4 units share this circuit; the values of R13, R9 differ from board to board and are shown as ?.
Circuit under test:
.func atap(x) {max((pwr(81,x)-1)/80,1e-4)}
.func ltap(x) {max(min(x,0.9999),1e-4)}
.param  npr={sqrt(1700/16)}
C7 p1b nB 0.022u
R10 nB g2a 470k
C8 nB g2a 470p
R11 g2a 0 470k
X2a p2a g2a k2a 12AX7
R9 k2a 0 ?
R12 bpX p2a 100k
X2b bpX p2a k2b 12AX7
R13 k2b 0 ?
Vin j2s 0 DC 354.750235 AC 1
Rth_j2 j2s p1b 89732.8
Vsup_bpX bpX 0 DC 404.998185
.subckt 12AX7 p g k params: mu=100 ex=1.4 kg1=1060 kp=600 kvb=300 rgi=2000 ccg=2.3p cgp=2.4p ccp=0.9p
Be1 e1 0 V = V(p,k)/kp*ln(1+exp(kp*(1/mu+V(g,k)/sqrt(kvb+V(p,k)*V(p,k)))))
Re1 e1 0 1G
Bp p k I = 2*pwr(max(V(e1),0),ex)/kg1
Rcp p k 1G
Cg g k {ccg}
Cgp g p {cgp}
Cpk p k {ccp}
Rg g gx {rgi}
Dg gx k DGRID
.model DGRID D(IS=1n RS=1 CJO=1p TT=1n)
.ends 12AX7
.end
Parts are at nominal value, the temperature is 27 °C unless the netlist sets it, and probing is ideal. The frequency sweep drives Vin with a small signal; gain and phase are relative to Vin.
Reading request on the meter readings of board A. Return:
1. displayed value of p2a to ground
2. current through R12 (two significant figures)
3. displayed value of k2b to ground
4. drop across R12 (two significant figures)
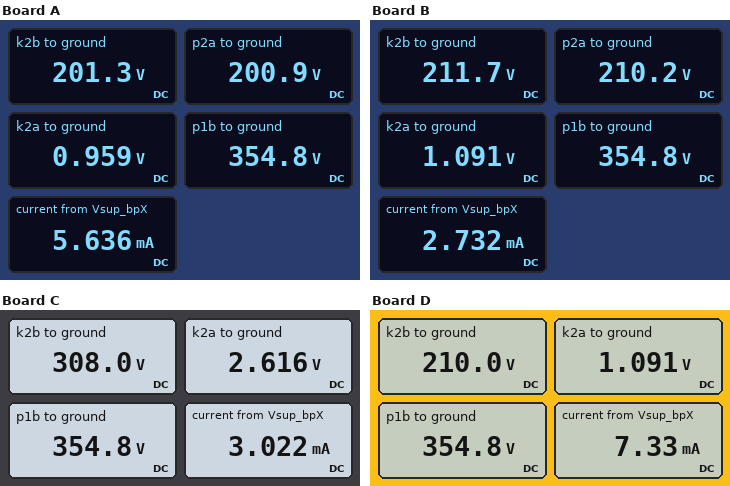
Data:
200.9 V
2.0 mA
201.3 V
200 V
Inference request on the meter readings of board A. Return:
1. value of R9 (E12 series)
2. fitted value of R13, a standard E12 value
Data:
470 Ω
56 kΩ
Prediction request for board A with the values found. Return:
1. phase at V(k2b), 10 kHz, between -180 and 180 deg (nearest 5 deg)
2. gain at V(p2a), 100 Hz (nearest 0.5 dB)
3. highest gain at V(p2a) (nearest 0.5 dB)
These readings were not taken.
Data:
155 deg
27.5 dB
31.0 dB
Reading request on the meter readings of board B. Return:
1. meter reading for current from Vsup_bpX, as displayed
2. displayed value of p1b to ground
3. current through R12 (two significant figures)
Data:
2.732 mA
354.8 V
1.9 mA
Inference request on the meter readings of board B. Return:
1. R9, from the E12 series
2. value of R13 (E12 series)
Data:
560 Ω
270 kΩ
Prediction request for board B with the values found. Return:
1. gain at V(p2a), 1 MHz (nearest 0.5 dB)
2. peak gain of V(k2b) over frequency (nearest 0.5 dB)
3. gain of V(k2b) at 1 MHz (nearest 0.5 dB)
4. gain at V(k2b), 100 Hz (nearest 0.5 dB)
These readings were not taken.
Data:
-3.0 dB
30.5 dB
-3.5 dB
27.0 dB
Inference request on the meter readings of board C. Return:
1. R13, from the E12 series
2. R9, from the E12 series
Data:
150 kΩ
2.7 kΩ
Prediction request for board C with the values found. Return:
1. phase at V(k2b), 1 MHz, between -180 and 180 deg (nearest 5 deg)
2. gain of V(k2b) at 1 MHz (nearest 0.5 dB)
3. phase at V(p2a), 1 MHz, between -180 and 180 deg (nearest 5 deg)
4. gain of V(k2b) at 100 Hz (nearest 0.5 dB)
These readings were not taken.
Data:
85 deg
-4.0 dB
85 deg
20.0 dB
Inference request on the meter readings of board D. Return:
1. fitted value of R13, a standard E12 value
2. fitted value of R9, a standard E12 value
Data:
39 kΩ
560 Ω
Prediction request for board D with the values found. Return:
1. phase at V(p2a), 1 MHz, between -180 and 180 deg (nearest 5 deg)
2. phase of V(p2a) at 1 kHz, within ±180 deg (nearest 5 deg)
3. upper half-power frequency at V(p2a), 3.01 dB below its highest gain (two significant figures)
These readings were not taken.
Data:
90 deg
-170 deg
22 kHz
